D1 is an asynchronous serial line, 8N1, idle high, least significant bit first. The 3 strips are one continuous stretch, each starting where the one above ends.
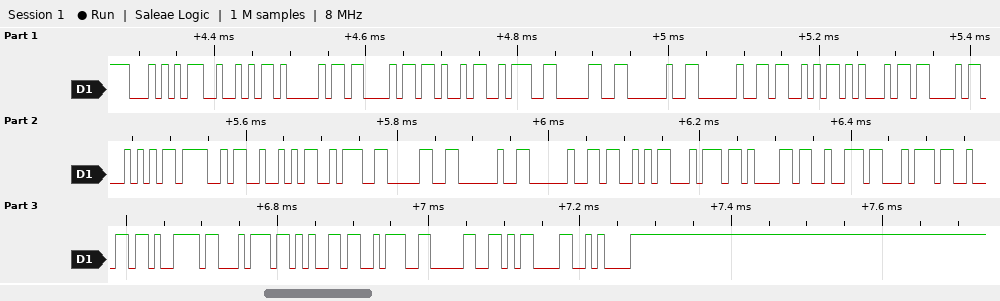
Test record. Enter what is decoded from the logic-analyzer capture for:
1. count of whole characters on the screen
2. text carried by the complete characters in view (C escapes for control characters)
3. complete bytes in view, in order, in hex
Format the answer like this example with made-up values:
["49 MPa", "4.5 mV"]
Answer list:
["32", "\"TRACK:0  SECTOR:0  Startbyte:0\\r\\n\"", "54 52 41 43 4B 3A 30 20 20 53 45 43 54 4F 52 3A 30 20 20 53 74 61 72 74 62 79 74 65 3A 30 0D 0A"]
